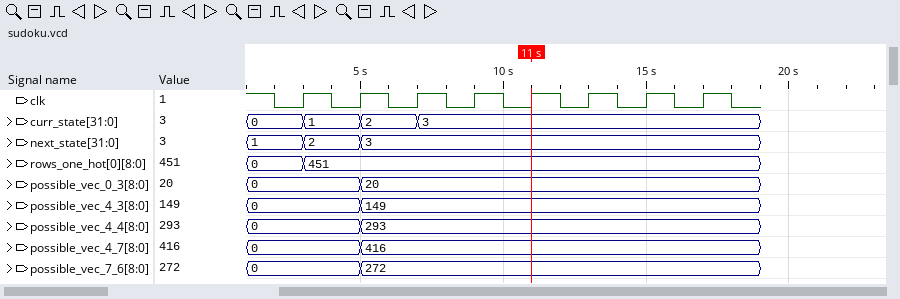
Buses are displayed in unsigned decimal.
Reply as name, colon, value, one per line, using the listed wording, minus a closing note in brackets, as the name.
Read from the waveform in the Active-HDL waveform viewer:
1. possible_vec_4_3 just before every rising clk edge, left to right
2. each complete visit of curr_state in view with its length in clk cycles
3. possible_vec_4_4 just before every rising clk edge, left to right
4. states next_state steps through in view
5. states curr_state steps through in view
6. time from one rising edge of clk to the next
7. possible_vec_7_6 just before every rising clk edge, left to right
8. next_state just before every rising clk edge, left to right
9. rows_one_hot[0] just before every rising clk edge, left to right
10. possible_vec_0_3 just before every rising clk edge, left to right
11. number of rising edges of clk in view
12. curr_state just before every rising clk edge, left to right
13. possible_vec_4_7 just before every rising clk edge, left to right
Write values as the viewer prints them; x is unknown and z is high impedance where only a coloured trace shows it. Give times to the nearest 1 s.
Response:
possible_vec_4_3 just before every rising clk edge, left to right: 0, 0, 149, 149, 149, 149, 149, 149
each complete visit of curr_state in view with its length in clk cycles: 1: 1, 2: 1
possible_vec_4_4 just before every rising clk edge, left to right: 0, 0, 293, 293, 293, 293, 293, 293
states next_state steps through in view: 1, 2, 3
states curr_state steps through in view: 0, 1, 2, 3
time from one rising edge of clk to the next: 2 s
possible_vec_7_6 just before every rising clk edge, left to right: 0, 0, 272, 272, 272, 272, 272, 272
next_state just before every rising clk edge, left to right: 1, 2, 3, 3, 3, 3, 3, 3
rows_one_hot[0] just before every rising clk edge, left to right: 0, 451, 451, 451, 451, 451, 451, 451
possible_vec_0_3 just before every rising clk edge, left to right: 0, 0, 20, 20, 20, 20, 20, 20
number of rising edges of clk in view: 8
curr_state just before every rising clk edge, left to right: 0, 1, 2, 3, 3, 3, 3, 3
possible_vec_4_7 just before every rising clk edge, left to right: 0, 0, 416, 416, 416, 416, 416, 416
